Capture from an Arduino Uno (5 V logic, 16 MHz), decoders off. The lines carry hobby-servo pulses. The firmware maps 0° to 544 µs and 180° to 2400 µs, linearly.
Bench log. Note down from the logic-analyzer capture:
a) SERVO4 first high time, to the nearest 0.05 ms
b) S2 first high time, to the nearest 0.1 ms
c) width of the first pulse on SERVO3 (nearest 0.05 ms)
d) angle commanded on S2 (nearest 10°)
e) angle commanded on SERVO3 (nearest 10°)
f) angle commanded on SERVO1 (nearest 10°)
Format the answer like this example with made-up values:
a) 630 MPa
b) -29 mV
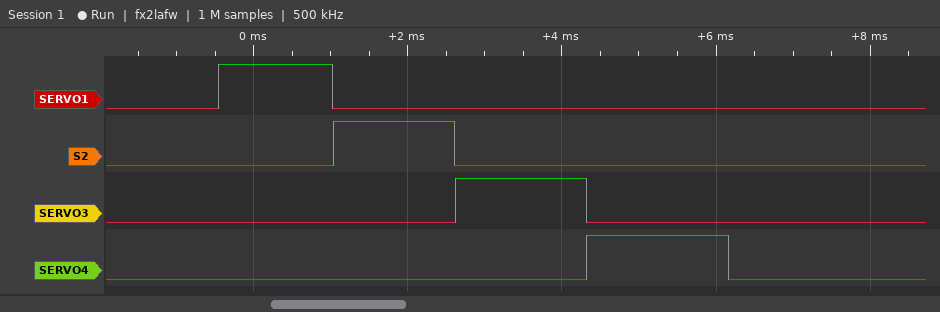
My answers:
a) 1.85 ms
b) 1.6 ms
c) 1.70 ms
d) 100°
e) 110°
f) 90°
